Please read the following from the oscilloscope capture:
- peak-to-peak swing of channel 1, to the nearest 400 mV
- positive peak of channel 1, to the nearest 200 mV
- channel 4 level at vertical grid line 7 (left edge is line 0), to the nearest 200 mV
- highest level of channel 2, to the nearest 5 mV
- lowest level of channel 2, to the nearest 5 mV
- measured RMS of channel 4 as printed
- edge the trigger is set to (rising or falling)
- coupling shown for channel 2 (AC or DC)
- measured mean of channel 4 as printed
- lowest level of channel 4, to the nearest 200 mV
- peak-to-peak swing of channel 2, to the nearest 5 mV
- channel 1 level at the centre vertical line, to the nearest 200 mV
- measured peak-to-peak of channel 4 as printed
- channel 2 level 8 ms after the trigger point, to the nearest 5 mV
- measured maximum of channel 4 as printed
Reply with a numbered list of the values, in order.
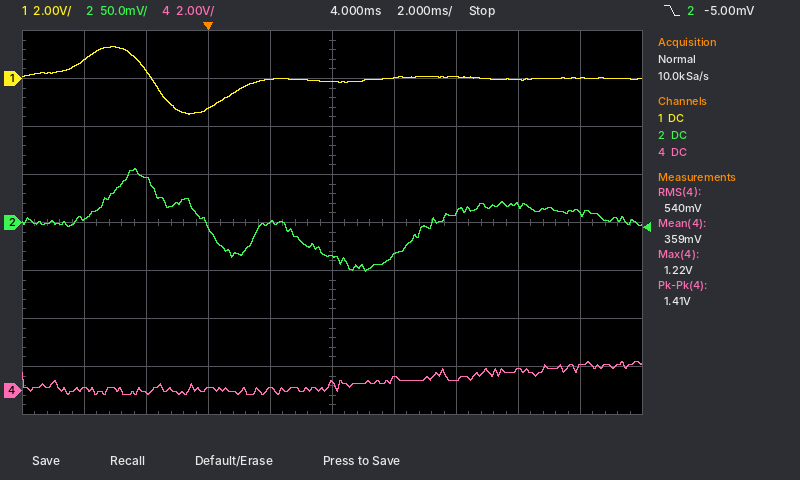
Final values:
1. 2.8 V
2. 1.4 V
3. 400 mV
4. 55 mV
5. -50 mV
6. 540 mV
7. falling
8. DC
9. 359 mV
10. -200 mV
11. 105 mV
12. -200 mV
13. 1.41 V
14. 10 mV
15. 1.22 V
